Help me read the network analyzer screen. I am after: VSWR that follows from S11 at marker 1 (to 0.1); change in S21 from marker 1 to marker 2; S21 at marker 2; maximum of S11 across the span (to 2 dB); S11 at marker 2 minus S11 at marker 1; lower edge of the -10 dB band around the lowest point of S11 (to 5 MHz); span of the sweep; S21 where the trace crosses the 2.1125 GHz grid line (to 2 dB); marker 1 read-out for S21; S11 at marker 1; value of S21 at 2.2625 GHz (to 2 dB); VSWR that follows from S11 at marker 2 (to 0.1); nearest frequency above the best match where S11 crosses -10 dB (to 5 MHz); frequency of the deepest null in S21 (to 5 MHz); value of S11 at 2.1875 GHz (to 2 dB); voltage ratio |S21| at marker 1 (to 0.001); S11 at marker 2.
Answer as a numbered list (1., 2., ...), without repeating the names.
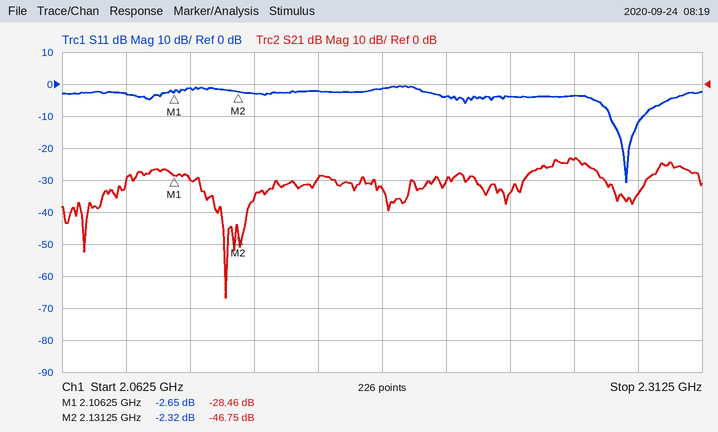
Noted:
1. 6.6
2. -18.29 dB
3. -46.75 dB
4. 0 dB
5. 0.33 dB
6. 2.275 GHz
7. 250 MHz
8. -30 dB
9. -28.46 dB
10. -2.65 dB
11. -24 dB
12. 7.5
13. 2.290 GHz
14. 2.125 GHz
15. -2 dB
16. 0.038
17. -2.32 dB
